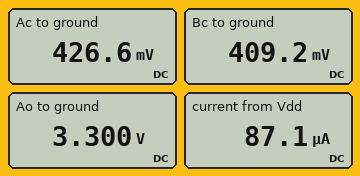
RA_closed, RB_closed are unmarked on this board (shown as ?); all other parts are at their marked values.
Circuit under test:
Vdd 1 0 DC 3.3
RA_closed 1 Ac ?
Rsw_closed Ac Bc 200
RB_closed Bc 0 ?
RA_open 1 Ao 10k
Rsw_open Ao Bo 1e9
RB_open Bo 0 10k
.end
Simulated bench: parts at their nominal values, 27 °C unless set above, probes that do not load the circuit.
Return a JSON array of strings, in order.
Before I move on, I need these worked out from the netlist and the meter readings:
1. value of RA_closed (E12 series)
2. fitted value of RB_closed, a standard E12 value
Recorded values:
["33 kΩ", "4.7 kΩ"]
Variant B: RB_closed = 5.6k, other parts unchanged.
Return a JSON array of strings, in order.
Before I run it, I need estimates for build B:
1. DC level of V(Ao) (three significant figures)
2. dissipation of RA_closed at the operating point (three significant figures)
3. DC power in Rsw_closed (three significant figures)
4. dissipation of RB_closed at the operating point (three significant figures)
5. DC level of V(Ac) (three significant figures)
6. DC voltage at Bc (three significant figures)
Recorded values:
["3.30 V", "239 µW", "1.45 µW", "40.5 µW", "493 mV", "476 mV"]
